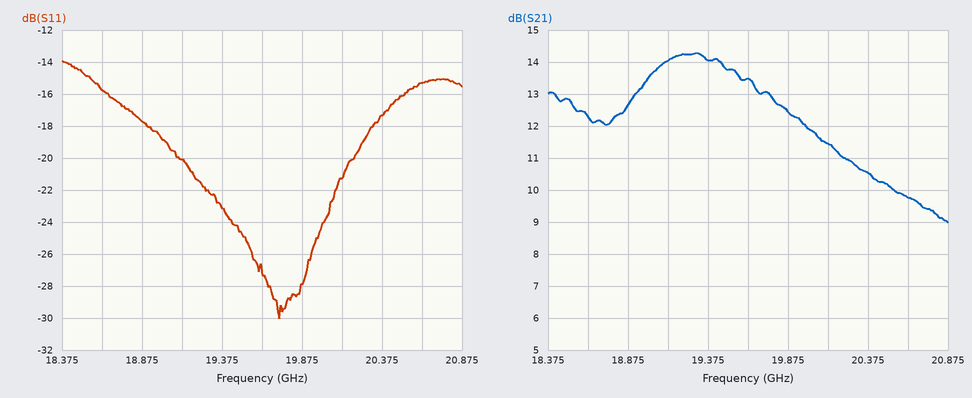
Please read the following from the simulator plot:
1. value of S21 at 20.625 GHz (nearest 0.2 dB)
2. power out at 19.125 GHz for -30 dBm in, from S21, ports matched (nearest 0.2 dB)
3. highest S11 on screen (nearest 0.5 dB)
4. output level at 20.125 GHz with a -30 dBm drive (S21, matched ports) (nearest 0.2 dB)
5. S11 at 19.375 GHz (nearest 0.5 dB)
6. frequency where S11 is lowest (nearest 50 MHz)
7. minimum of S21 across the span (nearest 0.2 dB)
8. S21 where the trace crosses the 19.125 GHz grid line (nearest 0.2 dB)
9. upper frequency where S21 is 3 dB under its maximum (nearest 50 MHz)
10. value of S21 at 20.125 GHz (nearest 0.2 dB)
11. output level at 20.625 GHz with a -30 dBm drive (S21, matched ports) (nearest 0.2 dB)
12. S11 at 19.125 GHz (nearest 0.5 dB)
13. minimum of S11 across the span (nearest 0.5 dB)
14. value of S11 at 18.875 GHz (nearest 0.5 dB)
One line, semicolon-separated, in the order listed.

9.8 dB; -16.0 dBm; -14.0 dB; -18.6 dBm; -23.0 dB; 19.75 GHz; 9.0 dB; 14.0 dB; 20.15 GHz; 11.4 dB; -20.2 dBm; -20.0 dB; -30.0 dB; -17.5 dB
